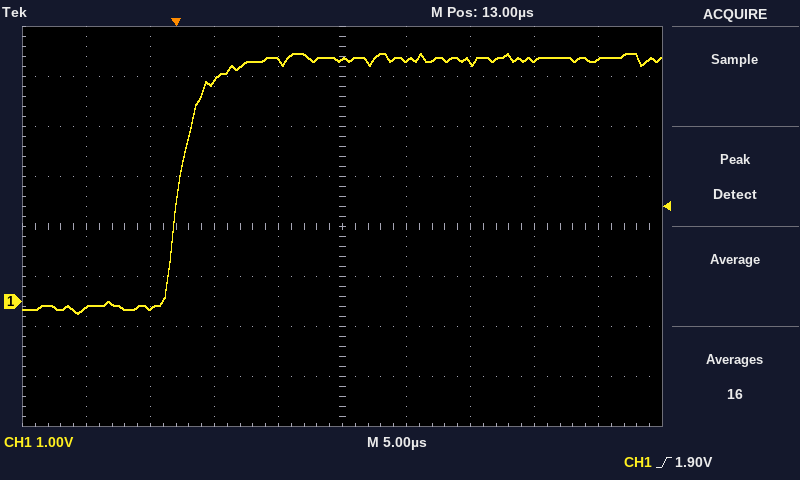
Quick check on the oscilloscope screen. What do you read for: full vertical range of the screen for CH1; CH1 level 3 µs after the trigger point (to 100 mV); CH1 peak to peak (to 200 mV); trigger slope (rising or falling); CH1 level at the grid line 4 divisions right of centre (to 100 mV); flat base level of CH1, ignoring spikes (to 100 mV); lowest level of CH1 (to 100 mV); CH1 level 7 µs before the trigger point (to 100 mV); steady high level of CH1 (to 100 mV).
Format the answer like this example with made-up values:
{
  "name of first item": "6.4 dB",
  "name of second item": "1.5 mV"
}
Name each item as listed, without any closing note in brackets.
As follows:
{
  "full vertical range of the screen for CH1": "8 V",
  "CH1 level 3 µs after the trigger point": "4.4 V",
  "CH1 peak to peak": "5.2 V",
  "trigger slope": "rising",
  "CH1 level at the grid line 4 divisions right of centre": "4.8 V",
  "flat base level of CH1, ignoring spikes": "-100 mV",
  "lowest level of CH1": "-200 mV",
  "CH1 level 7 µs before the trigger point": "-100 mV",
  "steady high level of CH1": "4.9 V"
}
